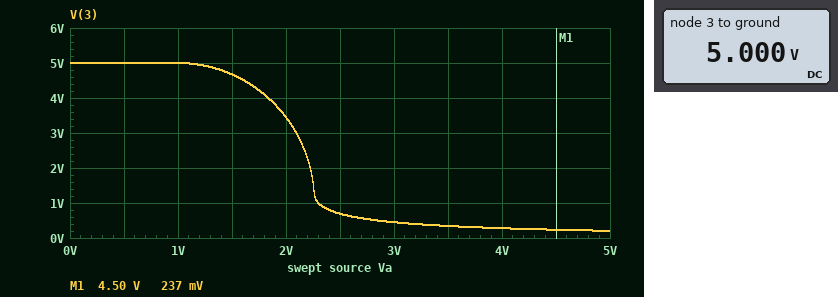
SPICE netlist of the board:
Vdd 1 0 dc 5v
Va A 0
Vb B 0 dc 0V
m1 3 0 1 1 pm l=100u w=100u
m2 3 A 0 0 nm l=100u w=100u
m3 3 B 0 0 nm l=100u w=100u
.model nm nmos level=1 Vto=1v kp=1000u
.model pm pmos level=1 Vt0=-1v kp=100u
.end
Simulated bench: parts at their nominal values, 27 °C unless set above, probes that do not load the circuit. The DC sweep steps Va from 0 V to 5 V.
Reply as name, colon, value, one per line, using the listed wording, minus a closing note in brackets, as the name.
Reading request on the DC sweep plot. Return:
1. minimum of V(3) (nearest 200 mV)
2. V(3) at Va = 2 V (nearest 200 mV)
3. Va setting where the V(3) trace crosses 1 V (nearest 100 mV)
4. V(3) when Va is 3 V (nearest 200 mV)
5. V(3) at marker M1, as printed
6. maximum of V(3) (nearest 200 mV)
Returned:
minimum of V(3): 200 mV
V(3) at Va = 2 V: 3.4 V
Va setting where the V(3) trace crosses 1 V: 2.3 V
V(3) when Va is 3 V: 400 mV
V(3) at marker M1, as printed: 237 mV
maximum of V(3): 5.0 V
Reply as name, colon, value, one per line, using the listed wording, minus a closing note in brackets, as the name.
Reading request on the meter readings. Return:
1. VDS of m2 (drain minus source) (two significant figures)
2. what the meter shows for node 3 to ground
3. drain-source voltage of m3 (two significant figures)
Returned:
VDS of m2 (drain minus source): 5.0 V
what the meter shows for node 3 to ground: 5.000 V
drain-source voltage of m3: 5.0 V
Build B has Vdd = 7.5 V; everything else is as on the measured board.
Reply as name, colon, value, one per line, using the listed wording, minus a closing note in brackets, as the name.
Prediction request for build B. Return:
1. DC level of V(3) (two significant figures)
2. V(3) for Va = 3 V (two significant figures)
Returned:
DC level of V(3): 7.5 V
V(3) for Va = 3 V: 2.5 V
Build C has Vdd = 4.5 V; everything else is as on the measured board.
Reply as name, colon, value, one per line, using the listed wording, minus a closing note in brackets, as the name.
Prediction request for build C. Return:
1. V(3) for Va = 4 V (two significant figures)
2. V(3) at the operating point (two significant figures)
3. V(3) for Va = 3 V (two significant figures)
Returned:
V(3) for Va = 4 V: 210 mV
V(3) at the operating point: 4.5 V
V(3) for Va = 3 V: 330 mV
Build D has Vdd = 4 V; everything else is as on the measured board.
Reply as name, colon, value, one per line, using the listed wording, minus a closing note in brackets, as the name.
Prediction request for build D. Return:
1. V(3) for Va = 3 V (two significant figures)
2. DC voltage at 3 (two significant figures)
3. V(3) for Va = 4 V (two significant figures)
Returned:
V(3) for Va = 3 V: 240 mV
DC voltage at 3: 4.0 V
V(3) for Va = 4 V: 150 mV
